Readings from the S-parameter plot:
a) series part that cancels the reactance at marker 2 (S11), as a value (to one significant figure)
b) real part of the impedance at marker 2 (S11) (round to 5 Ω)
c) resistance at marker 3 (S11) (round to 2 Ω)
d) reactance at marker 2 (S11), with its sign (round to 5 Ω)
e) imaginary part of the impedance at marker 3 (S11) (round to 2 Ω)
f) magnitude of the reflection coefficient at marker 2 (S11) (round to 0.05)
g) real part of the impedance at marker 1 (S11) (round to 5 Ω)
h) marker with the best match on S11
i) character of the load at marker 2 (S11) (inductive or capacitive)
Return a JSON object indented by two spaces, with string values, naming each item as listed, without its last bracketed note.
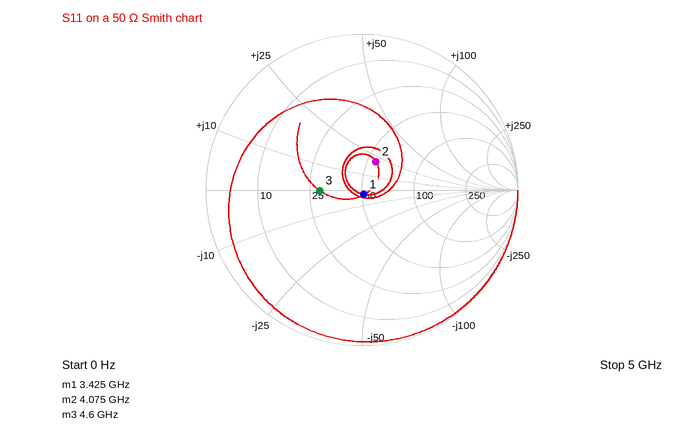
{
  "series part that cancels the reactance at marker 2 (S11), as a value": "2 pF",
  "real part of the impedance at marker 2 (S11)": "55 Ω",
  "resistance at marker 3 (S11)": "28 Ω",
  "reactance at marker 2 (S11), with its sign": "+20 Ω",
  "imaginary part of the impedance at marker 3 (S11)": "0 Ω",
  "magnitude of the reflection coefficient at marker 2 (S11)": "0.20",
  "real part of the impedance at marker 1 (S11)": "50 Ω",
  "marker with the best match on S11": "marker 1",
  "character of the load at marker 2 (S11)": "inductive"
}
